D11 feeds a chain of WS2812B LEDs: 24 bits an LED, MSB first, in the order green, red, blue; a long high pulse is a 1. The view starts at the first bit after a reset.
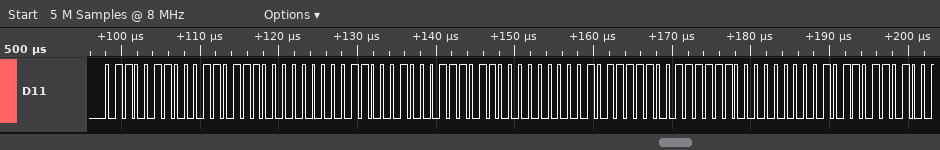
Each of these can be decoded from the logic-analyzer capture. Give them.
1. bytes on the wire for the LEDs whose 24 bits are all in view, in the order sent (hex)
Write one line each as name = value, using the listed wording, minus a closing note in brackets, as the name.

bytes on the wire for the LEDs whose 24 bits are all in view, in the order sent = 66 37 00 62 3B 00 5F 3F 00
